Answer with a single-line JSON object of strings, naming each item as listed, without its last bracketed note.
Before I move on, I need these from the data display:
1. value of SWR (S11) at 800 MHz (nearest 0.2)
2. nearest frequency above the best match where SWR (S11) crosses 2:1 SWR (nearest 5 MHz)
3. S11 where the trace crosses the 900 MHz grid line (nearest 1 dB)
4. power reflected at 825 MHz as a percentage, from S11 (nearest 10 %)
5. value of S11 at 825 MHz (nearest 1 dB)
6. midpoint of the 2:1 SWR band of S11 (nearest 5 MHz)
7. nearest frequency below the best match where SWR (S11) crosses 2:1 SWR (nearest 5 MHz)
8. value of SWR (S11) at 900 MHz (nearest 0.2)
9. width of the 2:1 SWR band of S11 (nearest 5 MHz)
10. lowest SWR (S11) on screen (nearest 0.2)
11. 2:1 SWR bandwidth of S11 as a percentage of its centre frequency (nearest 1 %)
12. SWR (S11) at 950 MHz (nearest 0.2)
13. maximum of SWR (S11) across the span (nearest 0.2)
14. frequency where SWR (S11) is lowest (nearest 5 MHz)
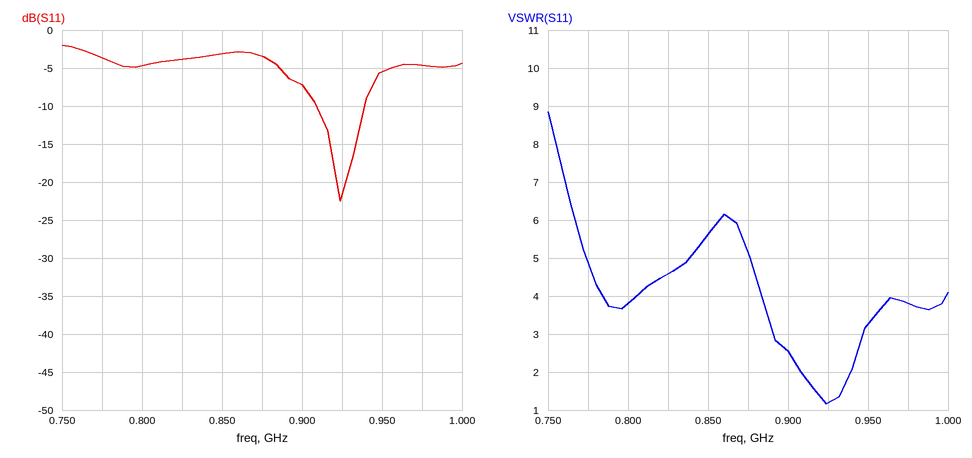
{"value of SWR (S11) at 800 MHz": "3.8", "nearest frequency above the best match where SWR (S11) crosses 2:1 SWR": "940 MHz", "S11 where the trace crosses the 900 MHz grid line": "-7 dB", "power reflected at 825 MHz as a percentage, from S11": "40 %", "value of S11 at 825 MHz": "-4 dB", "midpoint of the 2:1 SWR band of S11": "925 MHz", "nearest frequency below the best match where SWR (S11) crosses 2:1 SWR": "910 MHz", "value of SWR (S11) at 900 MHz": "2.6", "width of the 2:1 SWR band of S11": "30 MHz", "lowest SWR (S11) on screen": "1.2", "2:1 SWR bandwidth of S11 as a percentage of its centre frequency": "3 %", "SWR (S11) at 950 MHz": "3.2", "maximum of SWR (S11) across the span": "8.8", "frequency where SWR (S11) is lowest": "925 MHz"}
